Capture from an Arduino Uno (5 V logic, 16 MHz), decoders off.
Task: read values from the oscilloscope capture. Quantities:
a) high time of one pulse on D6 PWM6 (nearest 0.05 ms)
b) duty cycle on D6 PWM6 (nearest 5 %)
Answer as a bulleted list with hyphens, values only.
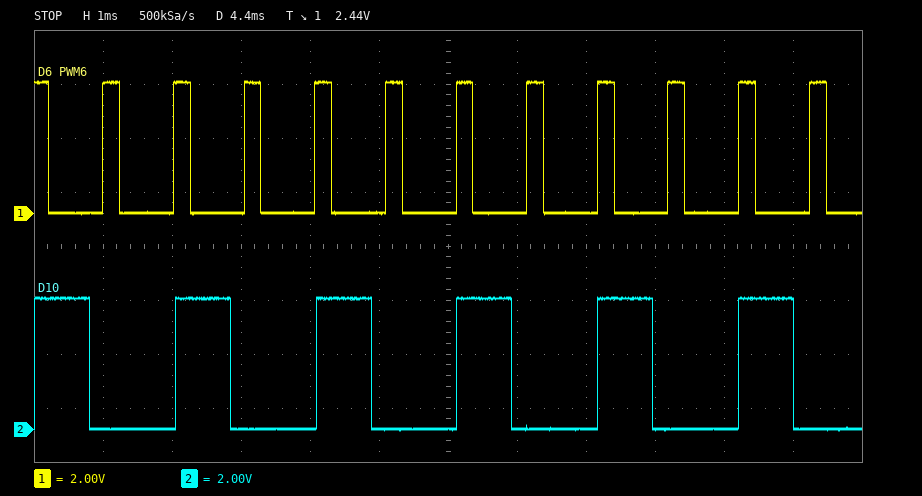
- 0.25 ms
- 25 %
